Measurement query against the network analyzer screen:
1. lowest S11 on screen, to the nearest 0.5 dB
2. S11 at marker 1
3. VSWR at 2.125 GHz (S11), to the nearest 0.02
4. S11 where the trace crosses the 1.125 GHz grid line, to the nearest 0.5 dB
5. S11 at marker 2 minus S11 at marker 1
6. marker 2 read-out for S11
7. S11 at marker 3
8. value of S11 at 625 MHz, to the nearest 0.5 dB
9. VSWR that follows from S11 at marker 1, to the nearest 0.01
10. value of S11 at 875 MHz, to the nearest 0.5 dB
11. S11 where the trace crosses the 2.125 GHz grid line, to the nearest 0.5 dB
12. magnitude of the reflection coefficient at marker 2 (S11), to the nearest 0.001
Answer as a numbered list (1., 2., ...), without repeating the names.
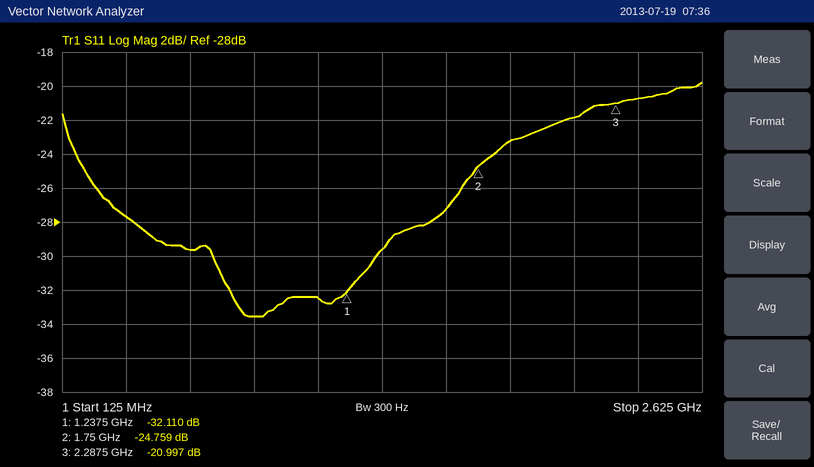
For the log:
1. -33.5 dB
2. -32.110 dB
3. 1.18
4. -32.5 dB
5. 7.351 dB
6. -24.759 dB
7. -20.997 dB
8. -29.5 dB
9. 1.05
10. -33.5 dB
11. -22.0 dB
12. 0.058
